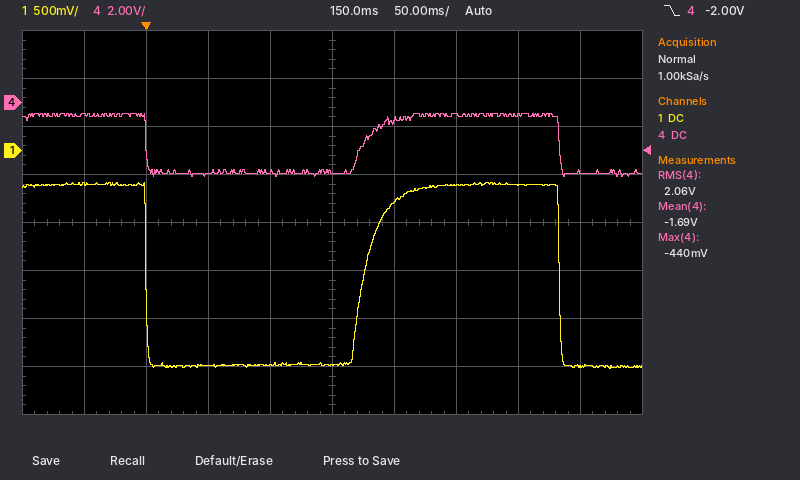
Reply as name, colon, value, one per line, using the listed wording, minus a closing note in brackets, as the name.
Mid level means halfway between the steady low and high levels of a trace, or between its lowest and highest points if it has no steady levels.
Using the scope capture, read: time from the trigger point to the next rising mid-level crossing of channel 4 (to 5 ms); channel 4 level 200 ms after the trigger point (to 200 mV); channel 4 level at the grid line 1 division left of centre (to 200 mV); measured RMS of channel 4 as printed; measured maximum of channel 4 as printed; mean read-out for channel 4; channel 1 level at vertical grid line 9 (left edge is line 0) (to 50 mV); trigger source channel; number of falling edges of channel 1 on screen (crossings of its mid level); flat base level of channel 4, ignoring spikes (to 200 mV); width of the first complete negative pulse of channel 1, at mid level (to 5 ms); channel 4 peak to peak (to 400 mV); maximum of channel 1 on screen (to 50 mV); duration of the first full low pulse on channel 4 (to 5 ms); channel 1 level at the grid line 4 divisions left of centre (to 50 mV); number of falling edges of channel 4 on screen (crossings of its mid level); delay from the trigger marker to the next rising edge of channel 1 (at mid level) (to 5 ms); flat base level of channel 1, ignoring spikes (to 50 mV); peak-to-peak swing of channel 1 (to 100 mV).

time from the trigger point to the next rising mid-level crossing of channel 4: 175 ms
channel 4 level 200 ms after the trigger point: -800 mV
channel 4 level at the grid line 1 division left of centre: -2.8 V
measured RMS of channel 4 as printed: 2.06 V
measured maximum of channel 4 as printed: -440 mV
mean read-out for channel 4: -1.69 V
channel 1 level at vertical grid line 9 (left edge is line 0): -2.25 V
trigger source channel: channel 4
number of falling edges of channel 1 on screen: 2
flat base level of channel 4, ignoring spikes: -3.0 V
width of the first complete negative pulse of channel 1, at mid level: 175 ms
channel 4 peak to peak: 2.8 V
maximum of channel 1 on screen: -350 mV
duration of the first full low pulse on channel 4: 175 ms
channel 1 level at the grid line 4 divisions left of centre: -350 mV
number of falling edges of channel 4 on screen: 2
delay from the trigger marker to the next rising edge of channel 1 (at mid level): 175 ms
flat base level of channel 1, ignoring spikes: -2.25 V
peak-to-peak swing of channel 1: 1.90 V
